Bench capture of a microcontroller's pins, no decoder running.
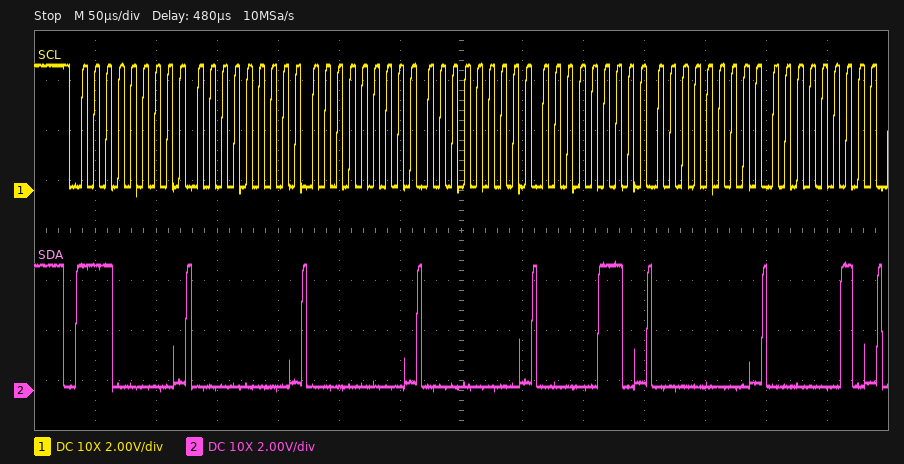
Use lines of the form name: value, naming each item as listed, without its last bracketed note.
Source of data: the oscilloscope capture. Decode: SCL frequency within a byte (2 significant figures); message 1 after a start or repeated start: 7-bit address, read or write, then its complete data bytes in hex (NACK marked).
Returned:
SCL frequency within a byte: 100 kHz
message 1 after a start or repeated start: 7-bit address, read or write, then its complete data bytes in hex: 0x70 write: 00 00 00 06 00 02
